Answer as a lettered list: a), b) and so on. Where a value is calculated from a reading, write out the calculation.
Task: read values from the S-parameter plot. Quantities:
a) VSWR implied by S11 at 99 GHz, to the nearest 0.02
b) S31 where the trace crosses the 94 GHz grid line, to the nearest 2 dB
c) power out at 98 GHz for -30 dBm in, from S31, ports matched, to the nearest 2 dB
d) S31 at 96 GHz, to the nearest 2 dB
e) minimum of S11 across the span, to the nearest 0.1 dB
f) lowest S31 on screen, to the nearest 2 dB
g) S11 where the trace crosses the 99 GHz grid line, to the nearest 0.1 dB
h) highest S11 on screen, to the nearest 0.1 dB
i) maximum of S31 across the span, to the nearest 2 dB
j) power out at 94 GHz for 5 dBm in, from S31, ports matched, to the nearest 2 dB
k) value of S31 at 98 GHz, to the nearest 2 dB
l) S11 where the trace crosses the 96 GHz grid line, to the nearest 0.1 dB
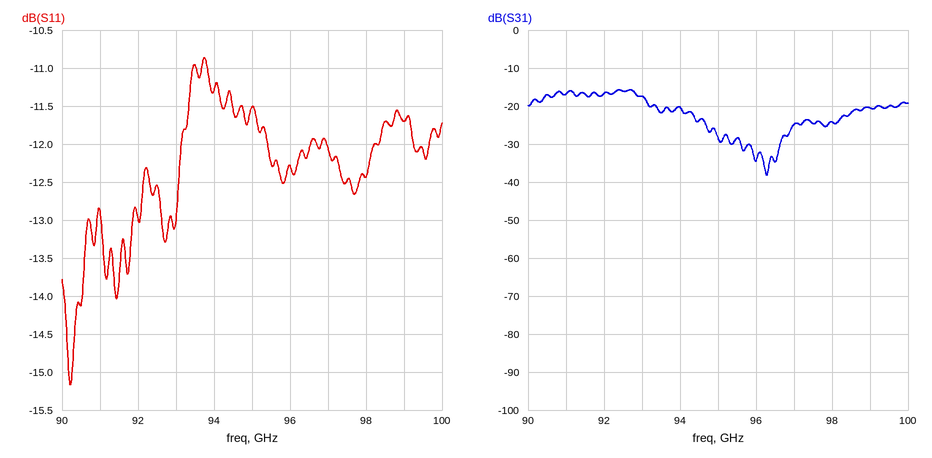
a) |Γ| = 10^(-11.7/20) = 0.2600; VSWR = (1 + 0.2600)/(1 − 0.2600) ≈ 1.70
b) -20 dB
c) -30 dBm + (-24 dB) = -54 dBm
d) -34 dB
e) -15.2 dB
f) -38 dB
g) -11.7 dB
h) -10.9 dB
i) -16 dB
j) 5 dBm + (-20 dB) = -16 dBm
k) -24 dB
l) -12.3 dB
